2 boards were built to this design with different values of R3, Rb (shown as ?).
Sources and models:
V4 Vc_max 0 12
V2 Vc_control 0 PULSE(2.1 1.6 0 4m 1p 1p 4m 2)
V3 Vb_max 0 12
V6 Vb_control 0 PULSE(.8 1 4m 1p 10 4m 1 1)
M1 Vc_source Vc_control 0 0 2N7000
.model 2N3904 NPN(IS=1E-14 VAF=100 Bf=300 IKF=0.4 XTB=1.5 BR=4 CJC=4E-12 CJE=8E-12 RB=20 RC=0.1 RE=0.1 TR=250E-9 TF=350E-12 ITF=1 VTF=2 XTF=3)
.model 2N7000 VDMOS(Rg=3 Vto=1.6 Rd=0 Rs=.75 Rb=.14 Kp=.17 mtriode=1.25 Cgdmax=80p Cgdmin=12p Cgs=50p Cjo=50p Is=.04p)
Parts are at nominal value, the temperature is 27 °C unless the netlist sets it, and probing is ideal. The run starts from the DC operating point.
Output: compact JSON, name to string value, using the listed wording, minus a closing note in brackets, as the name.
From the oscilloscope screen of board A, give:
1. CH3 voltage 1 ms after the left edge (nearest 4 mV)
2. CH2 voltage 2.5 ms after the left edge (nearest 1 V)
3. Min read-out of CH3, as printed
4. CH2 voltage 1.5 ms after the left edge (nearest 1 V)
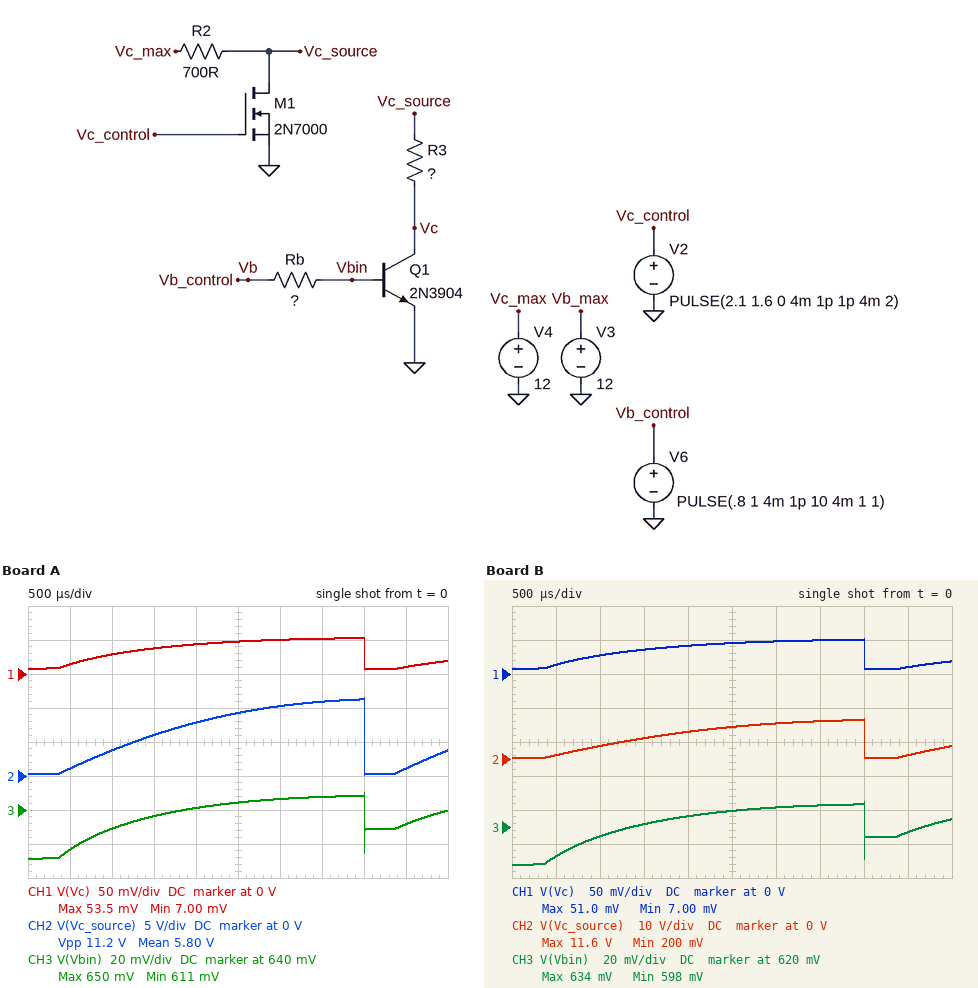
{"CH3 voltage 1 ms after the left edge": "628 mV", "CH2 voltage 2.5 ms after the left edge": "9 V", "Min read-out of CH3, as printed": "611 mV", "CH2 voltage 1.5 ms after the left edge": "6 V"}
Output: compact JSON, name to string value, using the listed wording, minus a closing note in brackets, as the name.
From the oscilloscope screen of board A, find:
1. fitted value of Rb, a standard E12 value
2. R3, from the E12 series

{"fitted value of Rb, a standard E12 value": "5.6 kΩ", "R3, from the E12 series": "18 kΩ"}
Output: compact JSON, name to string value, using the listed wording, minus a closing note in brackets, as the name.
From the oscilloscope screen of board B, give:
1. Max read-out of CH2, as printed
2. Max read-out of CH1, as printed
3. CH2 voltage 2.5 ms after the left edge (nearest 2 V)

{"Max read-out of CH2, as printed": "11.6 V", "Max read-out of CH1, as printed": "51.0 mV", "CH2 voltage 2.5 ms after the left edge": "10 V"}
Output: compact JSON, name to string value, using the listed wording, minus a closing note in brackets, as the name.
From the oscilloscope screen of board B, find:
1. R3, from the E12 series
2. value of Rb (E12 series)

{"R3, from the E12 series": "33 kΩ", "value of Rb": "10 kΩ"}
